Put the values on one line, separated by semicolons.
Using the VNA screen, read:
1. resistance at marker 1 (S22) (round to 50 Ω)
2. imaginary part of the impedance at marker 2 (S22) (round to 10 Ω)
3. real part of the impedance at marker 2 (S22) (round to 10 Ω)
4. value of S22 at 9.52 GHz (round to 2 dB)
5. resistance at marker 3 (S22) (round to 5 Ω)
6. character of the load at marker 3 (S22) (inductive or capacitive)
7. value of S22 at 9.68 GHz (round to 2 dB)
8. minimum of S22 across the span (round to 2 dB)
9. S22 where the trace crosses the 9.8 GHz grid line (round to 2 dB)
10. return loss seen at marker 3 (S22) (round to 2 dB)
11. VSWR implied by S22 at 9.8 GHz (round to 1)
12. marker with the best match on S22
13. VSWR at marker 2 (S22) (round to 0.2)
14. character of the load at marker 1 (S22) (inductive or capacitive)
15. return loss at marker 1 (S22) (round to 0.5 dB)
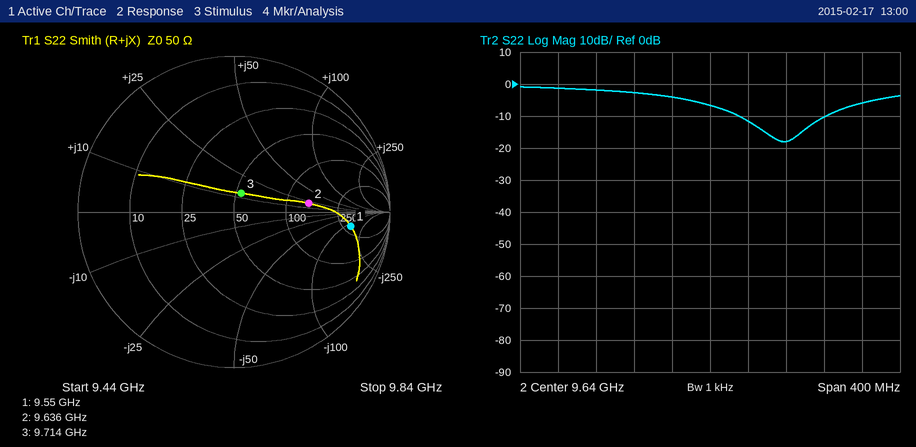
300 Ω; +20 Ω; 140 Ω; -2 dB; 55 Ω; inductive; -12 dB; -18 dB; -6 dB; 18 dB; 3; marker 3; 2.8; capacitive; 2.5 dB
